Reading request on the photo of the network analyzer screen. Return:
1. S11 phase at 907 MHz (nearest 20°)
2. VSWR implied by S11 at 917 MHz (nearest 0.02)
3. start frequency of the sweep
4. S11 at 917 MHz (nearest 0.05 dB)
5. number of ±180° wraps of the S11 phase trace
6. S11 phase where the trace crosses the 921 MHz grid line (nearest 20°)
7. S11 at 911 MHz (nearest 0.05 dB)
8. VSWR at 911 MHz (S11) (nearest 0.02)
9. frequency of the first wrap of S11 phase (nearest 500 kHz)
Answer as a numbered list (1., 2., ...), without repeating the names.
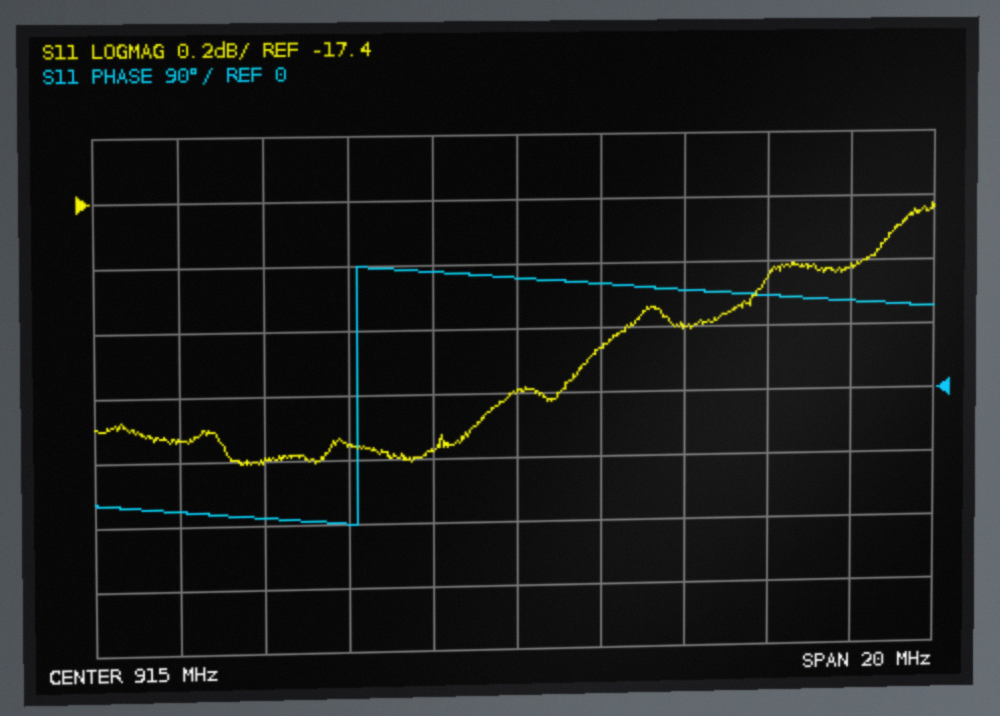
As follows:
1. -160°
2. 1.30
3. 905 MHz
4. -17.85 dB
5. 1
6. 140°
7. -18.15 dB
8. 1.28
9. 911.0 MHz
